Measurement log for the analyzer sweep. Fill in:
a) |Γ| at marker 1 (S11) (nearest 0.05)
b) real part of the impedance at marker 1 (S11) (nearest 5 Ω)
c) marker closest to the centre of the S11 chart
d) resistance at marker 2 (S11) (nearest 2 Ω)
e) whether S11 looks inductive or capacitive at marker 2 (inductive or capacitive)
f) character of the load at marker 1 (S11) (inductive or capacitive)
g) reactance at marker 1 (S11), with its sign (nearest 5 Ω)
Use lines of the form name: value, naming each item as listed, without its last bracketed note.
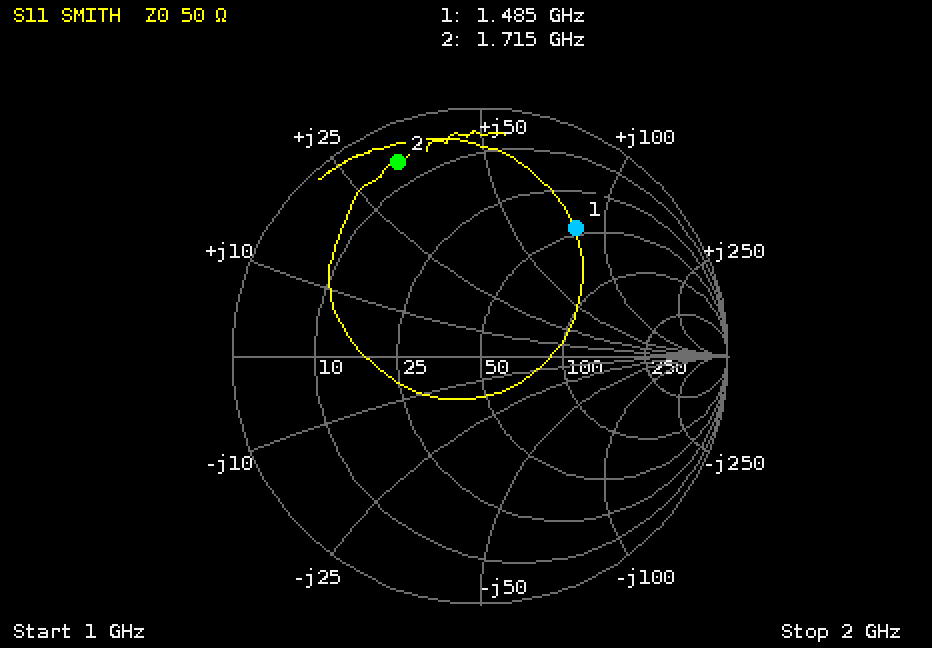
|Γ| at marker 1 (S11): 0.65
real part of the impedance at marker 1 (S11): 45 Ω
marker closest to the centre of the S11 chart: marker 1
resistance at marker 2 (S11): 6 Ω
whether S11 looks inductive or capacitive at marker 2: inductive
character of the load at marker 1 (S11): inductive
reactance at marker 1 (S11), with its sign: +80 Ω
